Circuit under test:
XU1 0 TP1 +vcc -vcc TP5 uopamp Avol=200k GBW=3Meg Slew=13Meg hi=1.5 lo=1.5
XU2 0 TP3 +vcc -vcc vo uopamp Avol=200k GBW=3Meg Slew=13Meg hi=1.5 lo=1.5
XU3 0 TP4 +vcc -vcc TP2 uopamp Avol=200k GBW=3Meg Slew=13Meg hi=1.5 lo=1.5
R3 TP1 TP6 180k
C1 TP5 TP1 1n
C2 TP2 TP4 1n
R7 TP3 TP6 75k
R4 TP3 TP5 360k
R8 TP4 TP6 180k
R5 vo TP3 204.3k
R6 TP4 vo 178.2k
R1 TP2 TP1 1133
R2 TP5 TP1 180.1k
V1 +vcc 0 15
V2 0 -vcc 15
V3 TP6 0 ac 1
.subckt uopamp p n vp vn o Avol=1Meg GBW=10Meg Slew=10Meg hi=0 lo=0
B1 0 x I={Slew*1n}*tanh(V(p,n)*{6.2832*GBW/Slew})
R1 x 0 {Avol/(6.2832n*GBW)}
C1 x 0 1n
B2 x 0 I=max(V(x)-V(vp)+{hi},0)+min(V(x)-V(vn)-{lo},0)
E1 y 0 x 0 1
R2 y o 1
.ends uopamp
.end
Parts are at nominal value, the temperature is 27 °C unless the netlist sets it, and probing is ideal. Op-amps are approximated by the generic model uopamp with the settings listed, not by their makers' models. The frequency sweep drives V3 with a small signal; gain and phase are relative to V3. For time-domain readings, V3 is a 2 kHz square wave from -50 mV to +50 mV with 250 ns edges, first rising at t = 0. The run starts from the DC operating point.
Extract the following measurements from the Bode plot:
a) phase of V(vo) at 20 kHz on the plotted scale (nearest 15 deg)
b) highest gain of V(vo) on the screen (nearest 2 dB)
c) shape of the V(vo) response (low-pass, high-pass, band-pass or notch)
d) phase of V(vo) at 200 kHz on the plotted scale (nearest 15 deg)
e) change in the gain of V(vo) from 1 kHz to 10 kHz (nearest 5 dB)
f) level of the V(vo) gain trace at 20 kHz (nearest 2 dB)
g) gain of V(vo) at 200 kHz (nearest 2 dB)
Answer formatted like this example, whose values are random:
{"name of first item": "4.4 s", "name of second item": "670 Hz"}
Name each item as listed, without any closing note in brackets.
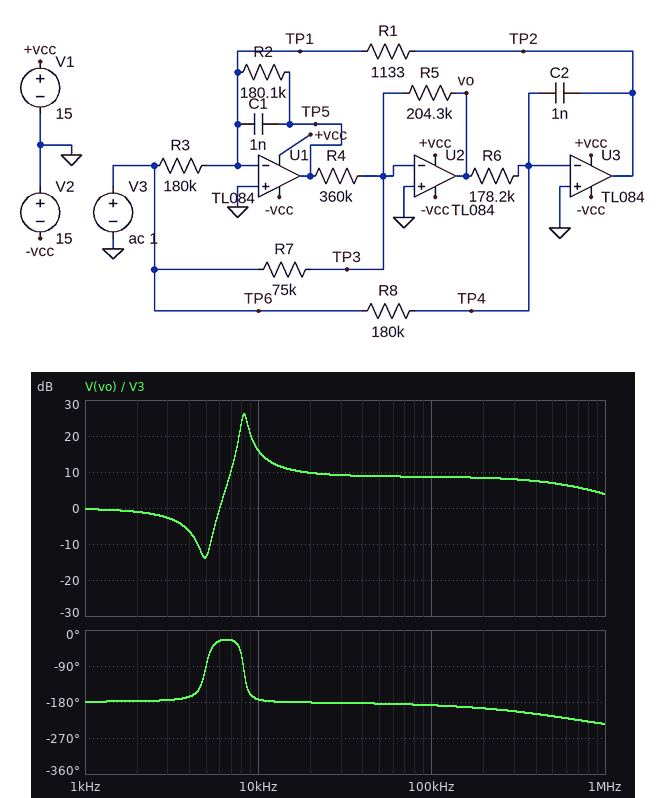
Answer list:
{"phase of V(vo) at 20 kHz on the plotted scale": "-180 deg", "highest gain of V(vo) on the screen": "26 dB", "shape of the V(vo) response": "band-pass", "phase of V(vo) at 200 kHz on the plotted scale": "-195 deg", "change in the gain of V(vo) from 1 kHz to 10 kHz": "15 dB", "level of the V(vo) gain trace at 20 kHz": "10 dB", "gain of V(vo) at 200 kHz": "8 dB"}
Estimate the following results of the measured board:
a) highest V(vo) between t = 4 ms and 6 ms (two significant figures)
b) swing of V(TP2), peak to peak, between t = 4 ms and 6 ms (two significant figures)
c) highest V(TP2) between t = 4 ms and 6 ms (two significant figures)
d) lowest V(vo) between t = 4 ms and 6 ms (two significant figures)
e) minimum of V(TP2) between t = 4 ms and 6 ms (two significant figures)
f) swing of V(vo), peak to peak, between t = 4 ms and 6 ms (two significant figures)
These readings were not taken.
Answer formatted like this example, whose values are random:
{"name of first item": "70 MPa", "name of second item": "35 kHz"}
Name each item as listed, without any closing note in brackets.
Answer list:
{"highest V(vo) between t = 4 ms and 6 ms": "160 mV", "swing of V(TP2), peak to peak, between t = 4 ms and 6 ms": "24 mV", "highest V(TP2) between t = 4 ms and 6 ms": "12 mV", "lowest V(vo) between t = 4 ms and 6 ms": "-160 mV", "minimum of V(TP2) between t = 4 ms and 6 ms": "-12 mV", "swing of V(vo), peak to peak, between t = 4 ms and 6 ms": "320 mV"}
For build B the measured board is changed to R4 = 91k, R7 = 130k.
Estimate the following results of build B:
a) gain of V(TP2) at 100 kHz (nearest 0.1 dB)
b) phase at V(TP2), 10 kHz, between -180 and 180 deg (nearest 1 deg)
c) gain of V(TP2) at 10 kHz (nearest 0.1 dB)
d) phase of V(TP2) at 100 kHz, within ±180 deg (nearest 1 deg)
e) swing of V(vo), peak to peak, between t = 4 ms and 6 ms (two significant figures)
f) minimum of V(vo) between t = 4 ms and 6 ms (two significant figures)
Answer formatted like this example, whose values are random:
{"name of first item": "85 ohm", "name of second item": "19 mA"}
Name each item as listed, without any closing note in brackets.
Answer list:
{"gain of V(TP2) at 100 kHz": "-45.3 dB", "phase at V(TP2), 10 kHz, between -180 and 180 deg": "100 deg", "gain of V(TP2) at 10 kHz": "-30.1 dB", "phase of V(TP2) at 100 kHz, within ±180 deg": "-115 deg", "swing of V(vo), peak to peak, between t = 4 ms and 6 ms": "170 mV", "minimum of V(vo) between t = 4 ms and 6 ms": "-83 mV"}
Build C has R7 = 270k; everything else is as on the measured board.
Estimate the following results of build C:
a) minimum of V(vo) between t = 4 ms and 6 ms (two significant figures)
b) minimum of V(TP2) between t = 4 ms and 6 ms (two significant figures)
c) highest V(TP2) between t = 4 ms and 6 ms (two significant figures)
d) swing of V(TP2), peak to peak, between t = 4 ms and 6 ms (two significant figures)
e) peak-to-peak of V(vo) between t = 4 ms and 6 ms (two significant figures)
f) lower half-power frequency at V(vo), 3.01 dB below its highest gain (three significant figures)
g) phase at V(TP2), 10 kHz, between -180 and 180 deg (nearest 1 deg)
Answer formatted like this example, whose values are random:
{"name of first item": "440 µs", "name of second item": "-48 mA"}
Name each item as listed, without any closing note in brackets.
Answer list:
{"minimum of V(vo) between t = 4 ms and 6 ms": "-63 mV", "minimum of V(TP2) between t = 4 ms and 6 ms": "-2.0 mV", "highest V(TP2) between t = 4 ms and 6 ms": "2.0 mV", "swing of V(TP2), peak to peak, between t = 4 ms and 6 ms": "4.0 mV", "peak-to-peak of V(vo) between t = 4 ms and 6 ms": "130 mV", "lower half-power frequency at V(vo), 3.01 dB below its highest gain": "7.52 kHz", "phase at V(TP2), 10 kHz, between -180 and 180 deg": "88 deg"}
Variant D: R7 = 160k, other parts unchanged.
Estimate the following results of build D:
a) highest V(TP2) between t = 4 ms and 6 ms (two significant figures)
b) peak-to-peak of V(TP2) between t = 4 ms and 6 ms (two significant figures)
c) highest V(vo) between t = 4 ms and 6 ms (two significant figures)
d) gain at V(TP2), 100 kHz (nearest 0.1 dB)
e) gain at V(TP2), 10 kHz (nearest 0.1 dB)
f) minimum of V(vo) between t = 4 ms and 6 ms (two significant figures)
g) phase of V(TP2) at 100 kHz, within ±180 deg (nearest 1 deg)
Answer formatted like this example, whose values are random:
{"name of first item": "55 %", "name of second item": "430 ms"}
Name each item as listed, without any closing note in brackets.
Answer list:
{"highest V(TP2) between t = 4 ms and 6 ms": "1.8 mV", "peak-to-peak of V(TP2) between t = 4 ms and 6 ms": "3.6 mV", "highest V(vo) between t = 4 ms and 6 ms": "68 mV", "gain at V(TP2), 100 kHz": "-51.4 dB", "gain at V(TP2), 10 kHz": "-22.2 dB", "minimum of V(vo) between t = 4 ms and 6 ms": "-68 mV", "phase of V(TP2) at 100 kHz, within ±180 deg": "-115 deg"}
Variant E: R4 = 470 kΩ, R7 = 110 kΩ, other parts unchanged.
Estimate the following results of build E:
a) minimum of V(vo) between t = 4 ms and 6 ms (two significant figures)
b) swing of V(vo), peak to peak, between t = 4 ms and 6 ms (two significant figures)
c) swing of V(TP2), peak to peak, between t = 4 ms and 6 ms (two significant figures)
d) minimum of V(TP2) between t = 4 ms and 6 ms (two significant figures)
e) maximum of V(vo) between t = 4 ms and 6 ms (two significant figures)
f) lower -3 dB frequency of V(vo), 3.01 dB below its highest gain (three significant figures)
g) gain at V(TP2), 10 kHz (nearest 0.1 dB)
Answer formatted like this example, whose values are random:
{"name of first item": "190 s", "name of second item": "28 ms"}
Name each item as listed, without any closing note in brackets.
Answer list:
{"minimum of V(vo) between t = 4 ms and 6 ms": "-110 mV", "swing of V(vo), peak to peak, between t = 4 ms and 6 ms": "220 mV", "swing of V(TP2), peak to peak, between t = 4 ms and 6 ms": "16 mV", "minimum of V(TP2) between t = 4 ms and 6 ms": "-8.2 mV", "maximum of V(vo) between t = 4 ms and 6 ms": "110 mV", "lower -3 dB frequency of V(vo), 3.01 dB below its highest gain": "6.95 kHz", "gain at V(TP2), 10 kHz": "-15.9 dB"}
